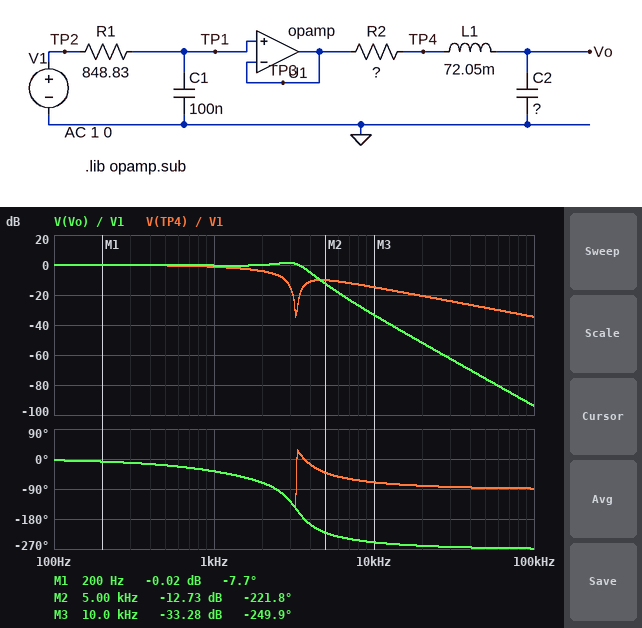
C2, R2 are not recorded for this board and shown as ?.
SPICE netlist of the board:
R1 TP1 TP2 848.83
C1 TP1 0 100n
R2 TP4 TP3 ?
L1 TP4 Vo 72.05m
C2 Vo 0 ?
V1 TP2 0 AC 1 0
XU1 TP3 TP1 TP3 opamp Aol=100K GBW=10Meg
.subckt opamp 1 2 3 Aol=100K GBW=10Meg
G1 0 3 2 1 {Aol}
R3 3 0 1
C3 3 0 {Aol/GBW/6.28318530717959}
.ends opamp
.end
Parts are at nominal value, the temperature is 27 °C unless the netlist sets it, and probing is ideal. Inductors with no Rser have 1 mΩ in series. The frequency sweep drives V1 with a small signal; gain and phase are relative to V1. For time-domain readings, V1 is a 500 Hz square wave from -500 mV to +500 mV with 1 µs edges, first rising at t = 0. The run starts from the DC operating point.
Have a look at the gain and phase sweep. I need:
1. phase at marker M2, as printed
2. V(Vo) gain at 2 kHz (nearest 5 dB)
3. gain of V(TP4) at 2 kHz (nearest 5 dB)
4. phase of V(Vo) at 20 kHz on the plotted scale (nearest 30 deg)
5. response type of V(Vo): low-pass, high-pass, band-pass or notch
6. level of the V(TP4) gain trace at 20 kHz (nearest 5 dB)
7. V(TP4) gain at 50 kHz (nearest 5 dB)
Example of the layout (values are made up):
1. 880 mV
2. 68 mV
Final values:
1. -221.8 deg
2. 0 dB
3. -5 dB
4. -270 deg
5. low-pass
6. -20 dB
7. -30 dB
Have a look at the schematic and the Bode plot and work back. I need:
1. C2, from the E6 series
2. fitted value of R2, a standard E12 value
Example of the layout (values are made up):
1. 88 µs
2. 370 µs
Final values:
1. 33 nF
2. 680 Ω
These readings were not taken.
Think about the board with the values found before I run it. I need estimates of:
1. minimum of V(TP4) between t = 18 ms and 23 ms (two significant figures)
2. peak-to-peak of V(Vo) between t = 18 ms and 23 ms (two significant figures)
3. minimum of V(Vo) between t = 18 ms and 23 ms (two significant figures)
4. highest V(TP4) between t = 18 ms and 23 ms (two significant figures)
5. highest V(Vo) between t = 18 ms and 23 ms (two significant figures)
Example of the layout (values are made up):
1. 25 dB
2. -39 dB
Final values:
1. -530 mV
2. 1.3 V
3. -630 mV
4. 530 mV
5. 630 mV
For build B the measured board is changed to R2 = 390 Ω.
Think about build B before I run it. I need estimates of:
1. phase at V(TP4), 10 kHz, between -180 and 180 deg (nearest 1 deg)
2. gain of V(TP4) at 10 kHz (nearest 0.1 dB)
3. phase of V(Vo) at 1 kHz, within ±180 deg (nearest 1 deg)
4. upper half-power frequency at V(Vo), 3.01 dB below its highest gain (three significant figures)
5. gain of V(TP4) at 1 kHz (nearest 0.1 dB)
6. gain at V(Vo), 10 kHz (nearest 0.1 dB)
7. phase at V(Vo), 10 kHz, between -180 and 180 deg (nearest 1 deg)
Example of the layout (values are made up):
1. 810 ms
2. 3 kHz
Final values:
1. -74 deg
2. -14.7 dB
3. -33 deg
4. 3.55 kHz
5. -1.1 dB
6. -33.2 dB
7. 106 deg
